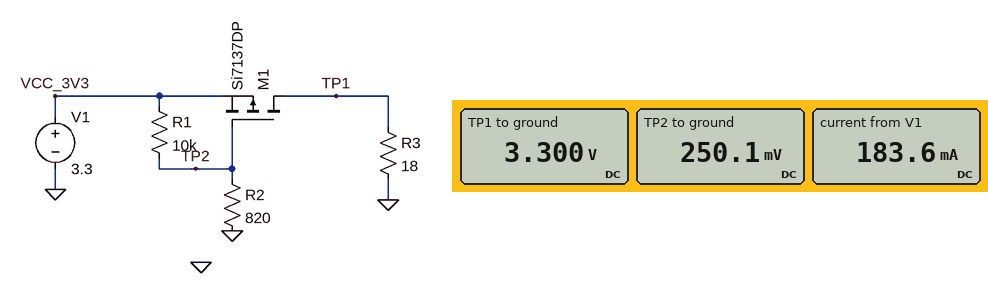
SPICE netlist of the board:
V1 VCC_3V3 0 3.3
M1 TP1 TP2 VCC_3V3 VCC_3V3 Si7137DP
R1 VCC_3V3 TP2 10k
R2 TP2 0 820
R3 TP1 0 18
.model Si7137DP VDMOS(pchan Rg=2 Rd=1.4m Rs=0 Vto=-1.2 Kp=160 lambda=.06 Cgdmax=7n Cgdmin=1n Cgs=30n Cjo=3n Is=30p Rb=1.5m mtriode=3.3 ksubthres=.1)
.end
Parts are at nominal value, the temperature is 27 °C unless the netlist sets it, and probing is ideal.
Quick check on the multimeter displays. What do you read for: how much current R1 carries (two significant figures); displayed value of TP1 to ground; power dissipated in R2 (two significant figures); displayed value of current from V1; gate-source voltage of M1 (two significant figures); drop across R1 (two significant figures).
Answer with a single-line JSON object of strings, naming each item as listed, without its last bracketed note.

{"how much current R1 carries": "300 µA", "displayed value of TP1 to ground": "3.300 V", "power dissipated in R2": "76 µW", "displayed value of current from V1": "183.6 mA", "gate-source voltage of M1": "-3.0 V", "drop across R1": "3.0 V"}
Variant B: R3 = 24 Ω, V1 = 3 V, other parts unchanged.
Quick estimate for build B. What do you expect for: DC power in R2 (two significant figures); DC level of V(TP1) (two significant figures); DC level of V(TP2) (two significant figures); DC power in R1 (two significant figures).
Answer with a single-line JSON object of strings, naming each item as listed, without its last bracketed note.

{"DC power in R2": "63 µW", "DC level of V(TP1)": "3.0 V", "DC level of V(TP2)": "230 mV", "DC power in R1": "770 µW"}
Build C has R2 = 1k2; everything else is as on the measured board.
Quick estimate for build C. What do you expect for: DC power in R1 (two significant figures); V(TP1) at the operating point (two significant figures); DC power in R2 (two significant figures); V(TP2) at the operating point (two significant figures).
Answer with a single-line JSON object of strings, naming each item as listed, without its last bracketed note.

{"DC power in R1": "870 µW", "V(TP1) at the operating point": "3.3 V", "DC power in R2": "100 µW", "V(TP2) at the operating point": "350 mV"}
